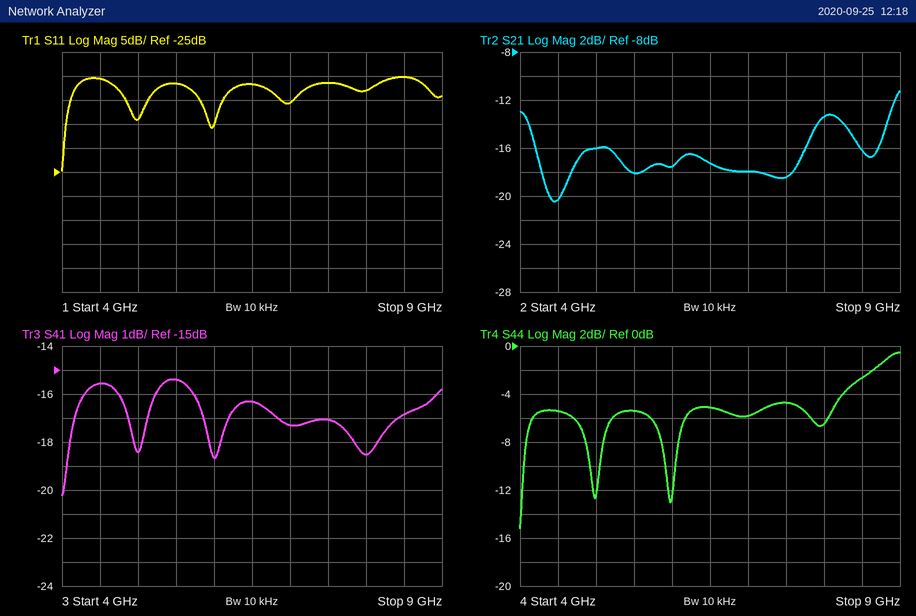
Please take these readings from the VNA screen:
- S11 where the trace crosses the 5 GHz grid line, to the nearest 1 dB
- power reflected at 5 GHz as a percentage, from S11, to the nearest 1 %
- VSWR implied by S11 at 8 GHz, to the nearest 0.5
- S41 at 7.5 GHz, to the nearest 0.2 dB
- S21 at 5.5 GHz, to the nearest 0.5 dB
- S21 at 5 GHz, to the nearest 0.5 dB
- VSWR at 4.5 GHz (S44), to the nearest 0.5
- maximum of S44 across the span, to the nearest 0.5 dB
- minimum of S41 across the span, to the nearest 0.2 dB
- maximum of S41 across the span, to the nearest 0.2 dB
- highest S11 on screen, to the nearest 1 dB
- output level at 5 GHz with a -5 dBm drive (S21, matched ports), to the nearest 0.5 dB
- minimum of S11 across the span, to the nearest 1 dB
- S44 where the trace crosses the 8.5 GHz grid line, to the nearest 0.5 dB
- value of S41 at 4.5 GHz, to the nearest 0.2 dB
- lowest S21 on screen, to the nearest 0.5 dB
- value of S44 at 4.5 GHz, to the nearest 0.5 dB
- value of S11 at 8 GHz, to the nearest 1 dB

-14 dB
4 %
2.5
-17.0 dB
-18.0 dB
-16.0 dB
3.5
-0.5 dB
-20.2 dB
-15.4 dB
-5 dB
-21.0 dBm
-25 dB
-2.5 dB
-15.6 dB
-20.5 dB
-5.5 dB
-8 dB
